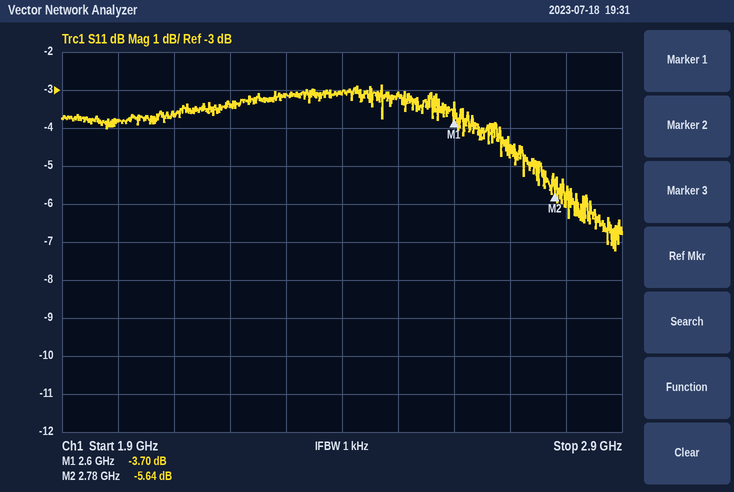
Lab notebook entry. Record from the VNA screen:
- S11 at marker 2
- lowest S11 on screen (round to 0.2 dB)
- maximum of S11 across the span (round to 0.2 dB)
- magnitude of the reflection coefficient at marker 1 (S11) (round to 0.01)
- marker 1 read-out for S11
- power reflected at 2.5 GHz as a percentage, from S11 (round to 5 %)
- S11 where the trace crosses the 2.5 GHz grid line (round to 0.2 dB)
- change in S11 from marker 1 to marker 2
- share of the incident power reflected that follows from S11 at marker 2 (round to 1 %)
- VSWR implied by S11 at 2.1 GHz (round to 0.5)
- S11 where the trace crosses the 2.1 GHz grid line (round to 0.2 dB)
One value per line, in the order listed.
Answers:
-5.64 dB
-7.2 dB
-2.8 dB
0.65
-3.70 dB
50 %
-3.2 dB
-1.94 dB
27 %
5.0
-3.6 dB
